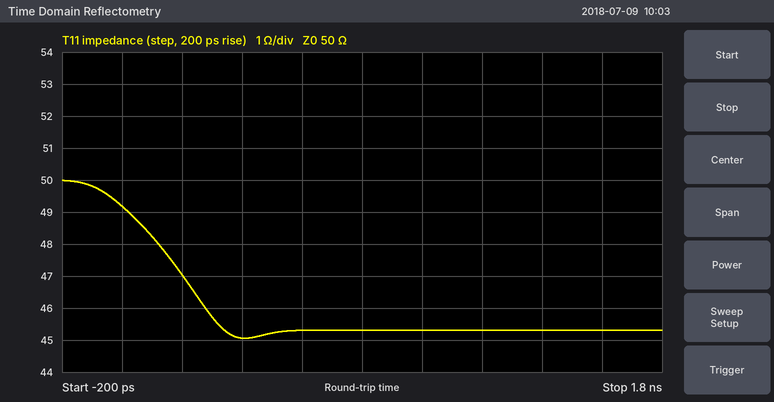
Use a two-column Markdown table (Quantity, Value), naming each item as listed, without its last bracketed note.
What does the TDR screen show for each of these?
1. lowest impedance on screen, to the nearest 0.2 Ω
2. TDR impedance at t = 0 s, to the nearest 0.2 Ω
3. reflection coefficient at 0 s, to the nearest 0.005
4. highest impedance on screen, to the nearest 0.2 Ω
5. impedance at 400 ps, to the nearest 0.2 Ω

| Quantity | Value |
|---|---|
| lowest impedance on screen, to the nearest 0.2 Ω | 45.0 Ω |
| TDR impedance at t = 0 s, to the nearest 0.2 Ω | 49.2 Ω |
| reflection coefficient at 0 s, to the nearest 0.005 | -0.010 |
| highest impedance on screen, to the nearest 0.2 Ω | 50.0 Ω |
| impedance at 400 ps, to the nearest 0.2 Ω | 45.0 Ω |
